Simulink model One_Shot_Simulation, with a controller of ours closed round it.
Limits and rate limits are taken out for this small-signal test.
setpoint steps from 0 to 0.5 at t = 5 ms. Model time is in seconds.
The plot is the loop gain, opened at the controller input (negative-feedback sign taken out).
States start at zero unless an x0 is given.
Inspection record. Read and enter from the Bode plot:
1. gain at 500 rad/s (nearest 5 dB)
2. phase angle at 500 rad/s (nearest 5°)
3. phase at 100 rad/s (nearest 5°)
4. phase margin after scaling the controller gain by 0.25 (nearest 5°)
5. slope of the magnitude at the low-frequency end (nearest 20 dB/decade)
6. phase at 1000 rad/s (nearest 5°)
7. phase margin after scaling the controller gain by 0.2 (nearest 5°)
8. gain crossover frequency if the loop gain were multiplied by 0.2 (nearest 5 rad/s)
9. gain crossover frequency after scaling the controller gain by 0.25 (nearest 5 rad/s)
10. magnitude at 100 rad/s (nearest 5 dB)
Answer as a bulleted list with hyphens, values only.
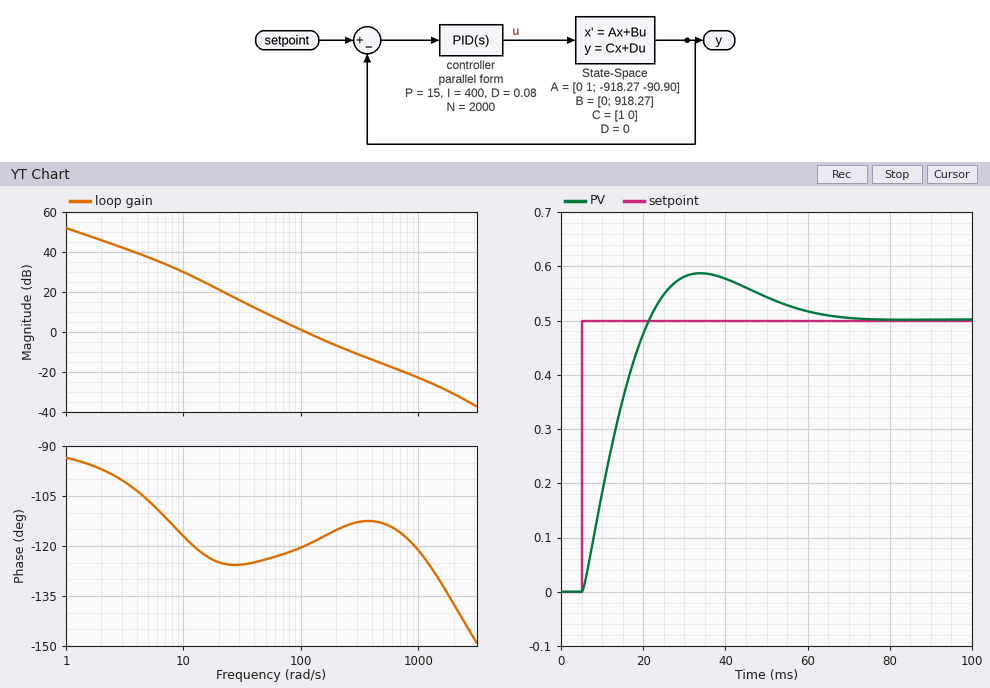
- -15 dB
- -115°
- -120°
- 55°
- -20 dB/decade
- -120°
- 55°
- 35 rad/s
- 40 rad/s
- 0 dB
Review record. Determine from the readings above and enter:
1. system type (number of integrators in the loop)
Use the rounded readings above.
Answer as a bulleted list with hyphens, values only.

- 1
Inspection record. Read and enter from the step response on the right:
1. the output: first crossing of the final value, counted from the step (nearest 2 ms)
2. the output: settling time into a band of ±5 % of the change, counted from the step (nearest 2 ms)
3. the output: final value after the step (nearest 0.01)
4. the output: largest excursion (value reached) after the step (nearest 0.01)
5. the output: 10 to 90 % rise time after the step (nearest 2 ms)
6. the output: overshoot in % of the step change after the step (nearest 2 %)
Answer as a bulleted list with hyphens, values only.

- 16 ms
- 52 ms
- 0.50
- 0.59
- 12 ms
- 18 %
